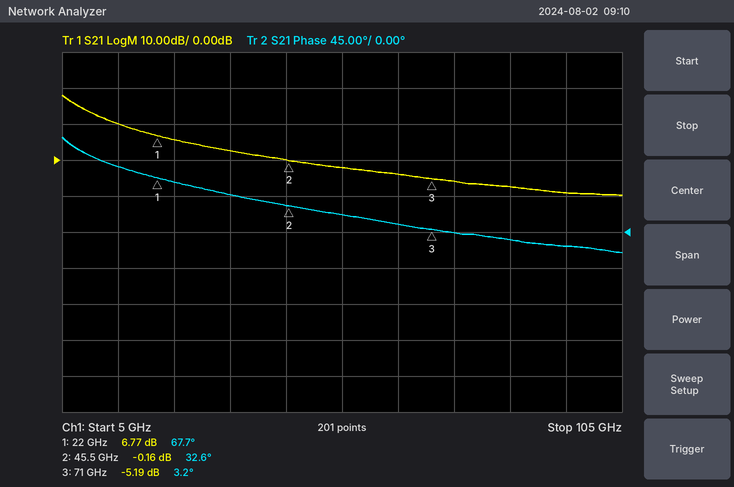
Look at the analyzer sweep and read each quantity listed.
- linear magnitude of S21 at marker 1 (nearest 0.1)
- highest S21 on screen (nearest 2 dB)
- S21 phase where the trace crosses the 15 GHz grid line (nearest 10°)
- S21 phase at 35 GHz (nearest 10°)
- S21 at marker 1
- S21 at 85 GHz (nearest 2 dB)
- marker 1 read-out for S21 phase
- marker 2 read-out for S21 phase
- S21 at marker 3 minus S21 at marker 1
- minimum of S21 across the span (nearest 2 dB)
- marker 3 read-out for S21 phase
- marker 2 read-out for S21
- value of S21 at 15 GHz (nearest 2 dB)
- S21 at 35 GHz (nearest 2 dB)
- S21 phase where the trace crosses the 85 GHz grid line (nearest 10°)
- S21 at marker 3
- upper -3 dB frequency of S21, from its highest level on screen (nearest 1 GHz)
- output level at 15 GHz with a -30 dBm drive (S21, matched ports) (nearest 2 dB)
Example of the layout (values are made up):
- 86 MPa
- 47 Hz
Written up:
- 2.2
- 18 dB
- 80°
- 50°
- 6.77 dB
- -8 dB
- 67.7°
- 32.6°
- -11.96 dB
- -10 dB
- 3.2°
- -0.16 dB
- 10 dB
- 2 dB
- -10°
- -5.19 dB
- 8 GHz
- -20 dBm
